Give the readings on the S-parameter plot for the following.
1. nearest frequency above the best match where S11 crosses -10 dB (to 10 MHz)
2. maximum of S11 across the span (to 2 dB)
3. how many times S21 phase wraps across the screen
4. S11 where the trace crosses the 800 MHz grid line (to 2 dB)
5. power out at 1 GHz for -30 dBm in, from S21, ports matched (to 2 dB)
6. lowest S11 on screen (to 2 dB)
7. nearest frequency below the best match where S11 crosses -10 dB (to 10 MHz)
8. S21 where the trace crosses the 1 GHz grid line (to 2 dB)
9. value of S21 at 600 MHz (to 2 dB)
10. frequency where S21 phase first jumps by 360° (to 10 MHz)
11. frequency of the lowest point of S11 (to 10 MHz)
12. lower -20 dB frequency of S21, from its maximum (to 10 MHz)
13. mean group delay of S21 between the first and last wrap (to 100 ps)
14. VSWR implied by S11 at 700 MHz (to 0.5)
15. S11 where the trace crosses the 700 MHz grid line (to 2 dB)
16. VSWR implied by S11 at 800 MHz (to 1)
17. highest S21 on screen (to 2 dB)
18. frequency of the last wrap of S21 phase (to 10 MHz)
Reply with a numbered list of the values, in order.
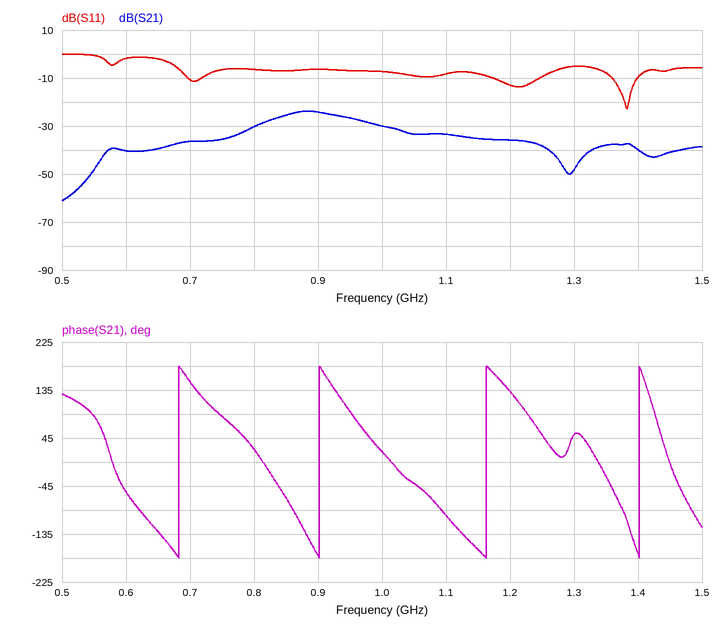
1. 1.40 GHz
2. 0 dB
3. 4
4. -6 dB
5. -60 dBm
6. -22 dB
7. 1.36 GHz
8. -30 dB
9. -40 dB
10. 680 MHz
11. 1.38 GHz
12. 560 MHz
13. 4.2 ns
14. 2.0
15. -10 dB
16. 3
17. -24 dB
18. 1.40 GHz
